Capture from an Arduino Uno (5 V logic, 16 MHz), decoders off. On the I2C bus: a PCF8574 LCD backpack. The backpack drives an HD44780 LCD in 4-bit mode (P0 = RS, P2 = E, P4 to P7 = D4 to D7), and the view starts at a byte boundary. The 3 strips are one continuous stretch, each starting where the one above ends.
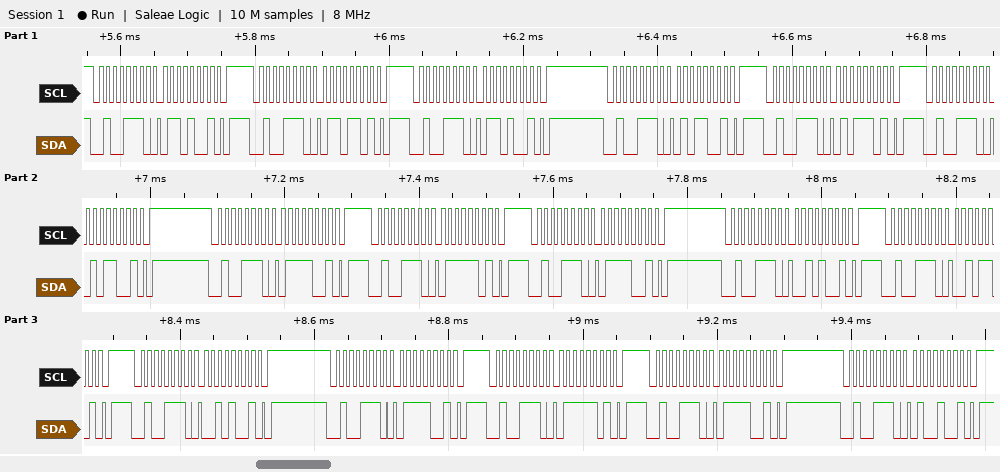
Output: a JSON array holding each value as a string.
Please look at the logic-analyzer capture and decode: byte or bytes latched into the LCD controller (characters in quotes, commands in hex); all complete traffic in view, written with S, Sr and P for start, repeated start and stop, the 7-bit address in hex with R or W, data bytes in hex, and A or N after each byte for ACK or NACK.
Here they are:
["'e' 'r'", "S 27W A 69 A P S 27W A 6D A P S 27W A 69 A P S 27W A 59 A P S 27W A 5D A P S 27W A 59 A P S 27W A 79 A P S 27W A 7D A P S 27W A 79 A P S 27W A 29 A P S 27W A 2D A P S 27W A 29 A P S 27W A 79 A P S 27W A 7D A P S 27W A 79 A P S 27W A 49 A P"]
